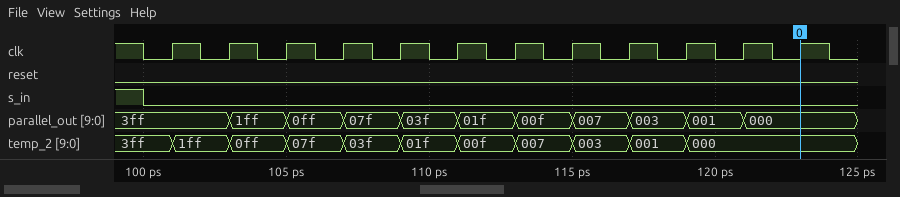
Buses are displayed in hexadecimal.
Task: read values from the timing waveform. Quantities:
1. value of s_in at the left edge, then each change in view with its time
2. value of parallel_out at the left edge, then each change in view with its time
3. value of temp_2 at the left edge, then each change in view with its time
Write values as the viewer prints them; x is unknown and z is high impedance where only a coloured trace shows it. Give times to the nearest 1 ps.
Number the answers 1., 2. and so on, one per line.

1. 1, 0 at 100 ps
2. 3ff, 1ff at 103 ps, 0ff at 105 ps, 07f at 107 ps, 03f at 109 ps, 01f at 111 ps, 00f at 113 ps, 007 at 115 ps, 003 at 117 ps, 001 at 119 ps, 000 at 121 ps
3. 3ff, 1ff at 101 ps, 0ff at 103 ps, 07f at 105 ps, 03f at 107 ps, 01f at 109 ps, 00f at 111 ps, 007 at 113 ps, 003 at 115 ps, 001 at 117 ps, 000 at 119 ps
